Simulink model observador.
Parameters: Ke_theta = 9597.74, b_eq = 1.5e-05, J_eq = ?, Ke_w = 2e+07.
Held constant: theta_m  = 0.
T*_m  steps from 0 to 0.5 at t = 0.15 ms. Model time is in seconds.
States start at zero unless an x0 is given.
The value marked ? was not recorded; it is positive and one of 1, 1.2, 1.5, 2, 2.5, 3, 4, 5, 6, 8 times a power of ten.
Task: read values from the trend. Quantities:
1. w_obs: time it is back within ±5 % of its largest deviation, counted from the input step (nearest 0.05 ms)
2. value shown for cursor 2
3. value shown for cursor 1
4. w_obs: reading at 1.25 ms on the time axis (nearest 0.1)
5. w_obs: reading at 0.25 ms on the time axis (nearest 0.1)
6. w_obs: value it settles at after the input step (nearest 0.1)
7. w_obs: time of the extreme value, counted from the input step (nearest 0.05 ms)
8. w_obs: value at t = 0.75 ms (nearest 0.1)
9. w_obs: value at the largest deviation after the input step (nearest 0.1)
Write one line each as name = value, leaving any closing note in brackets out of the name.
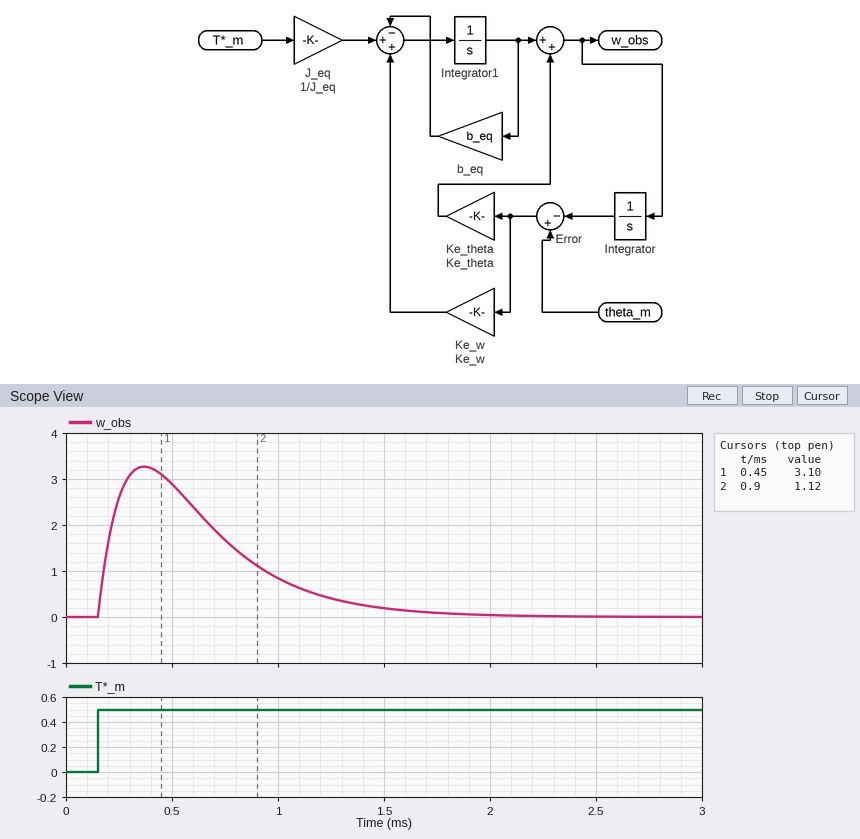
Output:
w_obs: time it is back within ±5 % of its largest deviation, counted from the input step = 1.40 ms
value shown for cursor 2 = 1.12
value shown for cursor 1 = 3.10
w_obs: reading at 1.25 ms on the time axis = 0.4
w_obs: reading at 0.25 ms on the time axis = 2.6
w_obs: value it settles at after the input step = 0.0
w_obs: time of the extreme value, counted from the input step = 0.20 ms
w_obs: value at t = 0.75 ms = 1.7
w_obs: value at the largest deviation after the input step = 3.3
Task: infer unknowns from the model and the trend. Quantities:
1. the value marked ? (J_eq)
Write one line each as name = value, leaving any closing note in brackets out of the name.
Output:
the value marked ? = 1.2e-05
